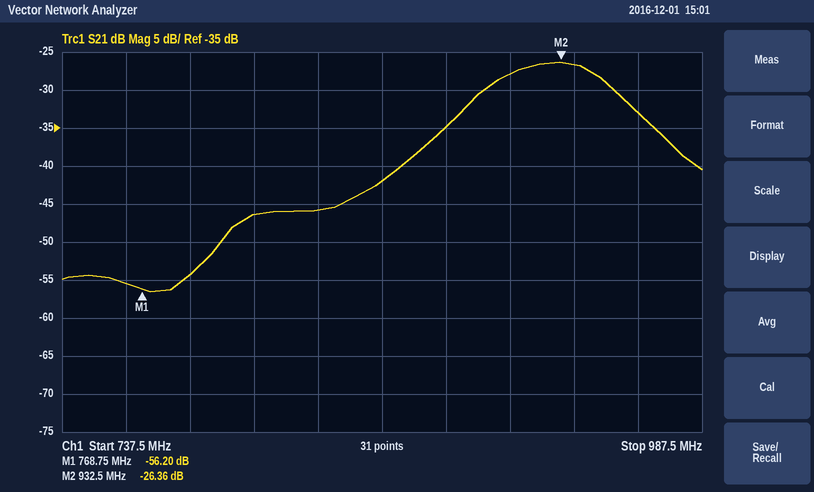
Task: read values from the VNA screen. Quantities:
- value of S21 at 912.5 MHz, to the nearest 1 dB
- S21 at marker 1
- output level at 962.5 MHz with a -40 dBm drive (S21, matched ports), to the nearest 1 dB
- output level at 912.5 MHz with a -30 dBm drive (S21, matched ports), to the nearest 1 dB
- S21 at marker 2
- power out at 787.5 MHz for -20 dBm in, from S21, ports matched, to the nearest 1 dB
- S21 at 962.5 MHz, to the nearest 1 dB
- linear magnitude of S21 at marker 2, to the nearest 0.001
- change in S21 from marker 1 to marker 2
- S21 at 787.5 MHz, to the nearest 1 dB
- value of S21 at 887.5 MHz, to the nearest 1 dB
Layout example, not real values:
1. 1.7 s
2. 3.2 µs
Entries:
1. -28 dB
2. -56.20 dB
3. -73 dBm
4. -58 dBm
5. -26.36 dB
6. -74 dBm
7. -33 dB
8. 0.048
9. 29.84 dB
10. -54 dB
11. -35 dB
